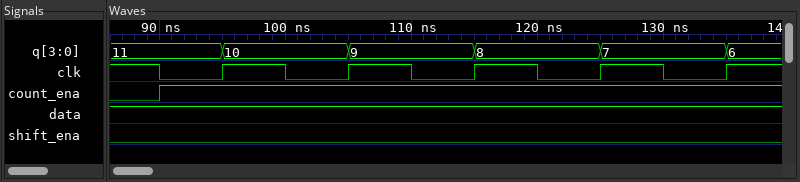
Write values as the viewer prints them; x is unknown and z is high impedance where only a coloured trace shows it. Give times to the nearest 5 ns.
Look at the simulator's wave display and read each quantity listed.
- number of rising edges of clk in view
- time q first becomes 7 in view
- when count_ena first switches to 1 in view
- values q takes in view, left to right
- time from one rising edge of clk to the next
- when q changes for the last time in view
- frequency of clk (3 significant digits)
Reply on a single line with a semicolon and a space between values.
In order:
5; 125 ns; 90 ns; 11, 10, 9, 8, 7, 6; 10 ns; 135 ns; 100 MHz
